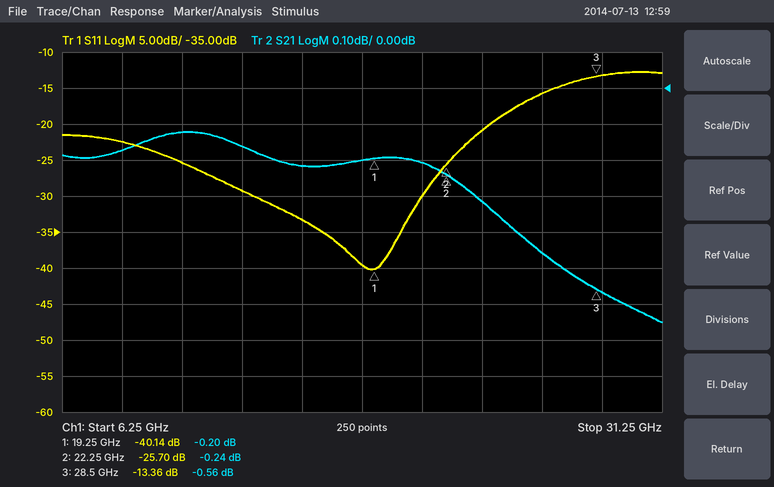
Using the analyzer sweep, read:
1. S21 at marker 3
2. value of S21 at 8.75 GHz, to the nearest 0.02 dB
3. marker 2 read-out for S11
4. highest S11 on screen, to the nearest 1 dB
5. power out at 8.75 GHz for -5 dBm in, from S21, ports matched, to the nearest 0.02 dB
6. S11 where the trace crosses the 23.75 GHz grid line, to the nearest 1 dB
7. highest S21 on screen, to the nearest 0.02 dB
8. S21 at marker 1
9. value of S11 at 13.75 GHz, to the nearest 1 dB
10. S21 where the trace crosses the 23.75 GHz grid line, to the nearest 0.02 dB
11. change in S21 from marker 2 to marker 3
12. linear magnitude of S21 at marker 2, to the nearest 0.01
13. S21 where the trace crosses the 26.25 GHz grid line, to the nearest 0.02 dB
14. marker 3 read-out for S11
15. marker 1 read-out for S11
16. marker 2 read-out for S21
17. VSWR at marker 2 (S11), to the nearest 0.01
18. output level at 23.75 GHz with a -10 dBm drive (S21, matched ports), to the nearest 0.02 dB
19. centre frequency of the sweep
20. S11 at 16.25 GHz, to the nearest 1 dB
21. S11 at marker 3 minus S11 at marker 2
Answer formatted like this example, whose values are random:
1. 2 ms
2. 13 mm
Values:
1. -0.56 dB
2. -0.18 dB
3. -25.70 dB
4. -13 dB
5. -5.18 dBm
6. -21 dB
7. -0.12 dB
8. -0.20 dB
9. -29 dB
10. -0.32 dB
11. -0.32 dB
12. 0.97
13. -0.46 dB
14. -13.36 dB
15. -40.14 dB
16. -0.24 dB
17. 1.11
18. -10.32 dBm
19. 18.75 GHz
20. -33 dB
21. 12.34 dB
